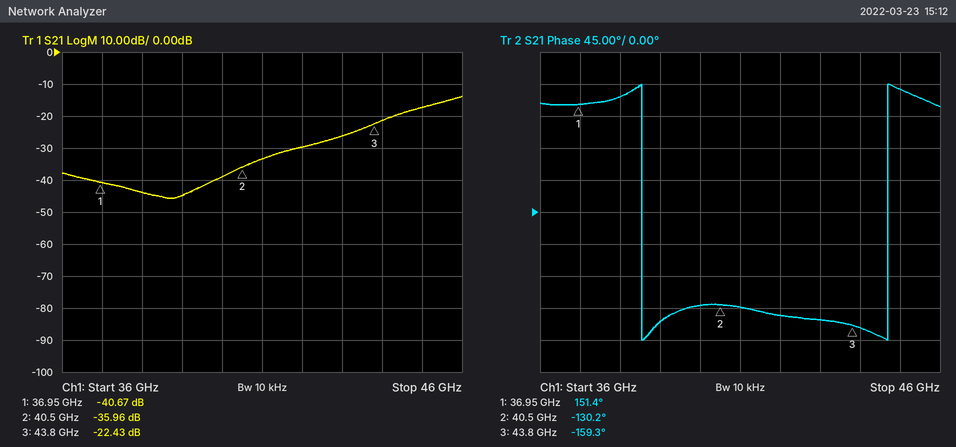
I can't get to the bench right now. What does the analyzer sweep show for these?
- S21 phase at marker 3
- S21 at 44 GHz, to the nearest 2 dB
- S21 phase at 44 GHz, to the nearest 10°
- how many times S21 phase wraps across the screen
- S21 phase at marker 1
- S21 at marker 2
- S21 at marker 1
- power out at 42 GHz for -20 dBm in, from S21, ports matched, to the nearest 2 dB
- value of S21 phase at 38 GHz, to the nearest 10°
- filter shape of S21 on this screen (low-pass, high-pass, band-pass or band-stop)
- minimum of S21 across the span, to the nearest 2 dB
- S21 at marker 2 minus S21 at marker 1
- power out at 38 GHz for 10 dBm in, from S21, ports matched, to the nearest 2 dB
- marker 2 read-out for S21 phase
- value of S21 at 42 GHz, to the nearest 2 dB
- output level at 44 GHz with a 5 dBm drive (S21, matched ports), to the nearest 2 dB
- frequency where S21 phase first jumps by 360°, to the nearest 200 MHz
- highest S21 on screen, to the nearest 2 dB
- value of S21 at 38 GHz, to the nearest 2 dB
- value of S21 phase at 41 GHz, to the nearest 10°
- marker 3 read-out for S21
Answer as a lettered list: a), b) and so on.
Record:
a) -159.3°
b) -22 dB
c) -160°
d) 2
e) 151.4°
f) -35.96 dB
g) -40.67 dB
h) -50 dBm
i) 160°
j) high-pass
k) -46 dB
l) 4.71 dB
m) -34 dBm
n) -130.2°
o) -30 dB
p) -16 dBm
q) 38.6 GHz
r) -14 dB
s) -44 dB
t) -130°
u) -22.43 dB
